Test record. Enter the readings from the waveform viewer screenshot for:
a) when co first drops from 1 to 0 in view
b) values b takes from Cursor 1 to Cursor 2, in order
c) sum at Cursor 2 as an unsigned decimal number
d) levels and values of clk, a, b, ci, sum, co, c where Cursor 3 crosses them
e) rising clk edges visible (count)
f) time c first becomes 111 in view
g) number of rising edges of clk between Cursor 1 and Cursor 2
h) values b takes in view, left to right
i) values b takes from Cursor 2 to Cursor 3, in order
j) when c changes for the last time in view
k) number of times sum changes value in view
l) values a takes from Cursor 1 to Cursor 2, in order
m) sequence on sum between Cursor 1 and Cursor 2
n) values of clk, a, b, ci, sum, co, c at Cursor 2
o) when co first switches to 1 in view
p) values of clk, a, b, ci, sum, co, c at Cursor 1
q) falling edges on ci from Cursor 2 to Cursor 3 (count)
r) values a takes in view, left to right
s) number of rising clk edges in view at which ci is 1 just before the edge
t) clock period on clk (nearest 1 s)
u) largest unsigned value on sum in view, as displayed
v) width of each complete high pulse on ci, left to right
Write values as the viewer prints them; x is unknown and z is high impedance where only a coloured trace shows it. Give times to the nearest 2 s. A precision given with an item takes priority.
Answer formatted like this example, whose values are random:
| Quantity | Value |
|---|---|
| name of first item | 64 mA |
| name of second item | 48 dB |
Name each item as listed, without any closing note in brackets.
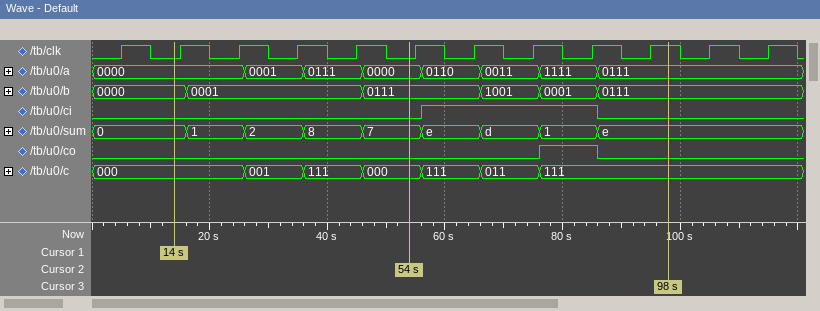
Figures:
| Quantity | Value |
|---|---|
| when co first drops from 1 to 0 in view | 86 s |
| values b takes from Cursor 1 to Cursor 2, in order | 0000, 0001, 0111 |
| sum at Cursor 2 as an unsigned decimal number | 7 |
| levels and values of clk, a, b, ci, sum, co, c where Cursor 3 crosses them | clk=1, a=0111, b=0111, ci=0, sum=e, co=0, c=111 |
| rising clk edges visible | 12 |
| time c first becomes 111 in view | 36 s |
| number of rising edges of clk between Cursor 1 and Cursor 2 | 4 |
| values b takes in view, left to right | 0000, 0001, 0111, 1001, 0001, 0111 |
| values b takes from Cursor 2 to Cursor 3, in order | 0111, 1001, 0001, 0111 |
| when c changes for the last time in view | 76 s |
| number of times sum changes value in view | 8 |
| values a takes from Cursor 1 to Cursor 2, in order | 0000, 0001, 0111, 0000 |
| sequence on sum between Cursor 1 and Cursor 2 | 0, 1, 2, 8, 7 |
| values of clk, a, b, ci, sum, co, c at Cursor 2 | clk=0, a=0000, b=0111, ci=0, sum=7, co=0, c=000 |
| when co first switches to 1 in view | 76 s |
| values of clk, a, b, ci, sum, co, c at Cursor 1 | clk=0, a=0000, b=0000, ci=0, sum=0, co=0, c=000 |
| falling edges on ci from Cursor 2 to Cursor 3 | 1 |
| values a takes in view, left to right | 0000, 0001, 0111, 0000, 0110, 0011, 1111, 0111 |
| number of rising clk edges in view at which ci is 1 just before the edge | 3 |
| clock period on clk | 10 s |
| largest unsigned value on sum in view, as displayed | e |
| width of each complete high pulse on ci, left to right | 30 s |
